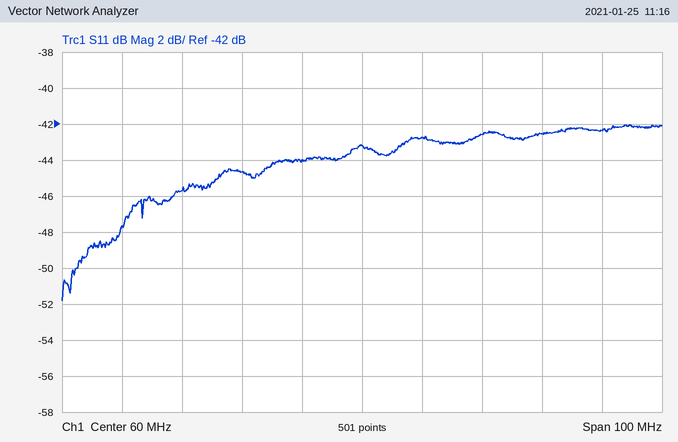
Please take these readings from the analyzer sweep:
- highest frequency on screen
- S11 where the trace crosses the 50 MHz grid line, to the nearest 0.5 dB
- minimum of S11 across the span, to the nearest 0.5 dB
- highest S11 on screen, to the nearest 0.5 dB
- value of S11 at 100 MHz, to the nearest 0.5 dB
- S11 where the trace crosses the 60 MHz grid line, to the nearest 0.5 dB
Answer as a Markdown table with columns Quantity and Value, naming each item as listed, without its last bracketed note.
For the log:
| Quantity | Value |
|---|---|
| highest frequency on screen | 110 MHz |
| S11 where the trace crosses the 50 MHz grid line, to the nearest 0.5 dB | -44.0 dB |
| minimum of S11 across the span, to the nearest 0.5 dB | -52.0 dB |
| highest S11 on screen, to the nearest 0.5 dB | -42.0 dB |
| value of S11 at 100 MHz, to the nearest 0.5 dB | -42.5 dB |
| S11 where the trace crosses the 60 MHz grid line, to the nearest 0.5 dB | -43.0 dB |
